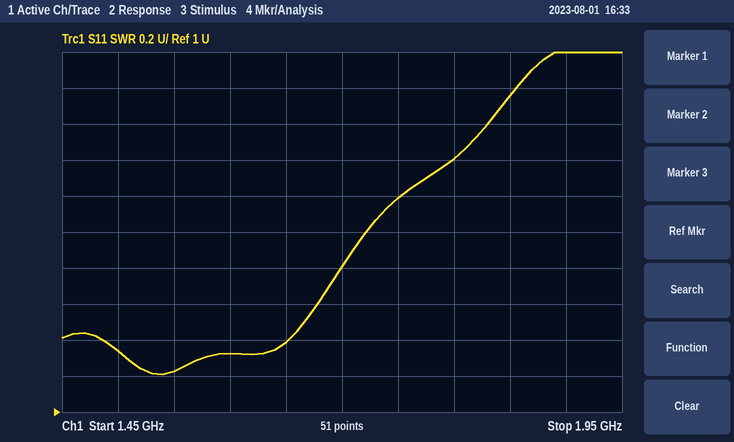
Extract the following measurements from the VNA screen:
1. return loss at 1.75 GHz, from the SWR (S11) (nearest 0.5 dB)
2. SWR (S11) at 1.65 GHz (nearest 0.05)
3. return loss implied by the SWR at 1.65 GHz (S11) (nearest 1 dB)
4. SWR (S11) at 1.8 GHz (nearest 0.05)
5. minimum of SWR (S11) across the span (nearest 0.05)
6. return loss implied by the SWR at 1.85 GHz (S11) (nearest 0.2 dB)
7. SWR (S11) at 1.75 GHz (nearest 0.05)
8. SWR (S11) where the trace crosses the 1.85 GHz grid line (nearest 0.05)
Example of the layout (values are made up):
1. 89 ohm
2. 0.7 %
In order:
1. 8.5 dB
2. 1.40
3. 16 dB
4. 2.40
5. 1.20
6. 6.6 dB
7. 2.20
8. 2.75
